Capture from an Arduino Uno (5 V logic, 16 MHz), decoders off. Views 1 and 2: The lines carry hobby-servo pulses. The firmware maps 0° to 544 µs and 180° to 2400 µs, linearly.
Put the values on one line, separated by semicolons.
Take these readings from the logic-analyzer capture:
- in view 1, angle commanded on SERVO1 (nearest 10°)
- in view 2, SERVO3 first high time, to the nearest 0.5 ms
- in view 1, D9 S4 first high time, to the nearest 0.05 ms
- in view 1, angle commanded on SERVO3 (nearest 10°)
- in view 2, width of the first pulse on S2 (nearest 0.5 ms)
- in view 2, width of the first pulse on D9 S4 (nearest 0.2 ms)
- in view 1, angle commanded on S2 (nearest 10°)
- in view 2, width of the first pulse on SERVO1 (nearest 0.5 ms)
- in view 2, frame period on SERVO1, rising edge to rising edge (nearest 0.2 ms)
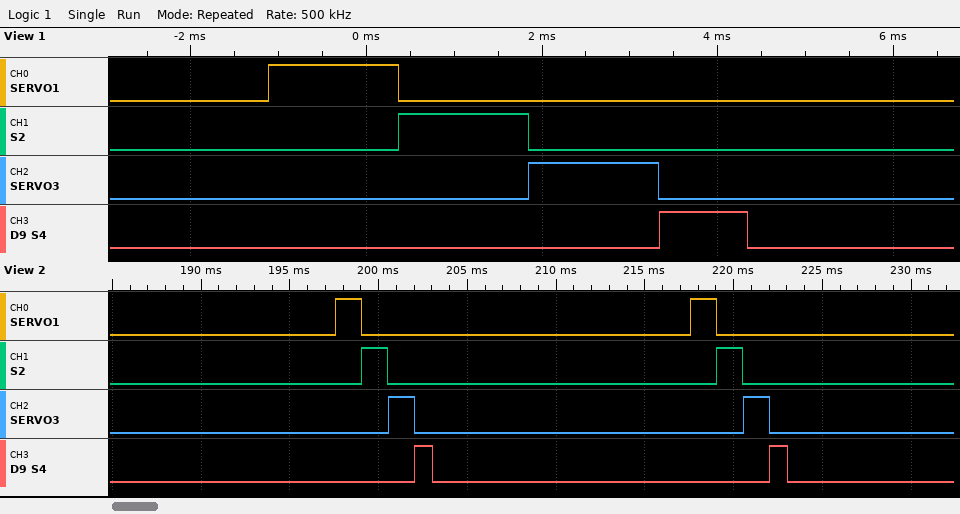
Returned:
90°; 1.5 ms; 1.00 ms; 90°; 1.5 ms; 1.0 ms; 90°; 1.5 ms; 20.0 ms
